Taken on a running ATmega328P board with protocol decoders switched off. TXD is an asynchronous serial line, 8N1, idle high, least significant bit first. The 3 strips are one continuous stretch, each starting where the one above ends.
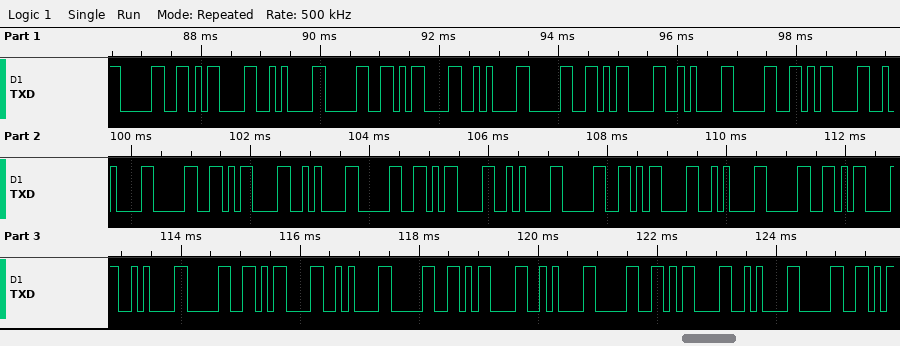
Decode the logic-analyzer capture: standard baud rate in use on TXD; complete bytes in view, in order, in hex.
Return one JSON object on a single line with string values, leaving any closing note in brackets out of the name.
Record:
{"standard baud rate in use on TXD": "9600 baud", "complete bytes in view, in order, in hex": "30 0D 0A 30 0D 0A 30 0D 0A 30 0D 0A 30 0D 0A 30 0D 0A 30 0D 0A 30 0D 0A 30 0D 0A 30 0D 0A 30 0D 0A 30"}
